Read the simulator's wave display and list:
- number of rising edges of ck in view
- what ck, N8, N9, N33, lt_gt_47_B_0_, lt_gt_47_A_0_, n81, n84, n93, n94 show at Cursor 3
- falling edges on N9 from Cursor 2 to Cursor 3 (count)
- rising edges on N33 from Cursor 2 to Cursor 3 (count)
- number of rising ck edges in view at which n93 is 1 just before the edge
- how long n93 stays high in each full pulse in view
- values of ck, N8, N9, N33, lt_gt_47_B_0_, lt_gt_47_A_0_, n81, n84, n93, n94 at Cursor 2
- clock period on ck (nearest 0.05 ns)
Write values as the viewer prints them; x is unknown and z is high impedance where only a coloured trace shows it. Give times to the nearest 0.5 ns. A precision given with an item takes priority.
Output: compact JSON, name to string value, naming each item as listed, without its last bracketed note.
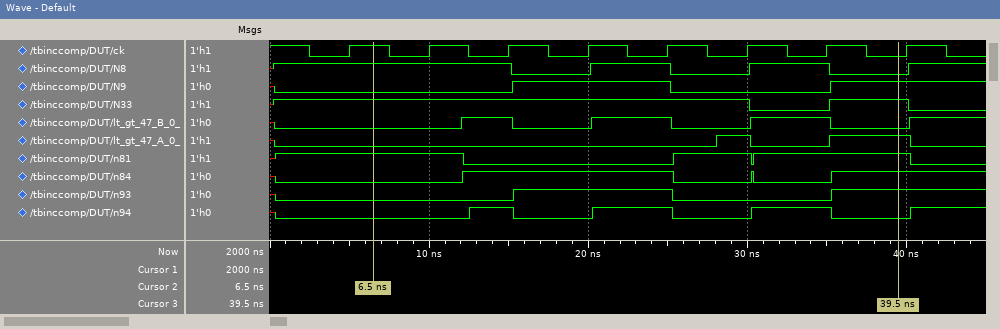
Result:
{"number of rising edges of ck in view": "8", "what ck, N8, N9, N33, lt_gt_47_B_0_, lt_gt_47_A_0_, n81, n84, n93, n94 show at Cursor 3": "ck=0, N8=0, N9=1, N33=1, lt_gt_47_B_0_=0, lt_gt_47_A_0_=1, n81=1, n84=1, n93=1, n94=0", "falling edges on N9 from Cursor 2 to Cursor 3": "1", "rising edges on N33 from Cursor 2 to Cursor 3": "1", "number of rising ck edges in view at which n93 is 1 just before the edge": "3", "how long n93 stays high in each full pulse in view": "10 ns", "values of ck, N8, N9, N33, lt_gt_47_B_0_, lt_gt_47_A_0_, n81, n84, n93, n94 at Cursor 2": "ck=1, N8=1, N9=0, N33=1, lt_gt_47_B_0_=0, lt_gt_47_A_0_=0, n81=1, n84=0, n93=0, n94=0", "clock period on ck": "5 ns"}
